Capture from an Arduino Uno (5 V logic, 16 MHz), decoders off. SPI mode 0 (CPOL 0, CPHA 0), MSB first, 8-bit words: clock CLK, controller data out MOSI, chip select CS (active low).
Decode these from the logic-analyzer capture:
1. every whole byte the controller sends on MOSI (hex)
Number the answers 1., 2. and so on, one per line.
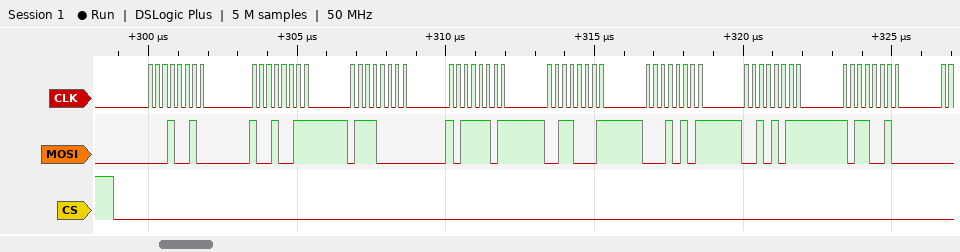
1. 12 93 70 BD 31 15 2B B2
